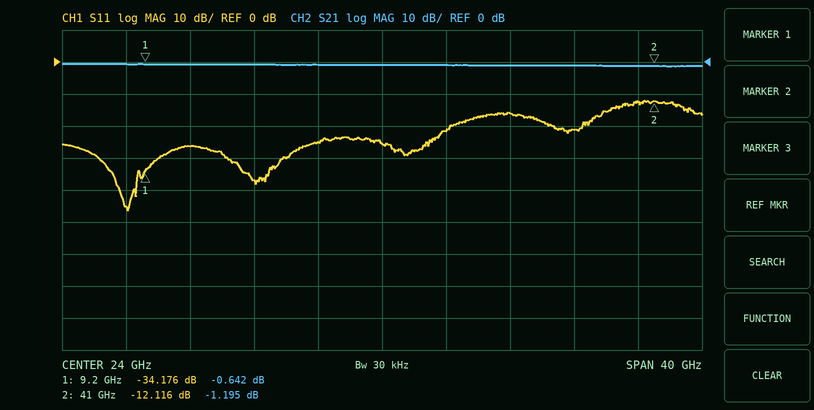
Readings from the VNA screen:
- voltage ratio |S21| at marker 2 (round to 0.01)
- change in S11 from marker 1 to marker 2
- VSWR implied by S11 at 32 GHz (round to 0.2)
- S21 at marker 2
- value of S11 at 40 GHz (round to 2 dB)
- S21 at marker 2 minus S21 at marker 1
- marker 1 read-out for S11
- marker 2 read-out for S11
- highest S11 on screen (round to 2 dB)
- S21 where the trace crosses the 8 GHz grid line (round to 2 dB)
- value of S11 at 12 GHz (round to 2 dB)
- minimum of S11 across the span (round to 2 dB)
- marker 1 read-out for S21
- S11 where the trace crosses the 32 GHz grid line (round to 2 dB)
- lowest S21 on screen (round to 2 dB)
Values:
0.87
22.060 dB
1.4
-1.195 dB
-12 dB
-0.553 dB
-34.176 dB
-12.116 dB
-12 dB
0 dB
-26 dB
-46 dB
-0.642 dB
-16 dB
-2 dB
